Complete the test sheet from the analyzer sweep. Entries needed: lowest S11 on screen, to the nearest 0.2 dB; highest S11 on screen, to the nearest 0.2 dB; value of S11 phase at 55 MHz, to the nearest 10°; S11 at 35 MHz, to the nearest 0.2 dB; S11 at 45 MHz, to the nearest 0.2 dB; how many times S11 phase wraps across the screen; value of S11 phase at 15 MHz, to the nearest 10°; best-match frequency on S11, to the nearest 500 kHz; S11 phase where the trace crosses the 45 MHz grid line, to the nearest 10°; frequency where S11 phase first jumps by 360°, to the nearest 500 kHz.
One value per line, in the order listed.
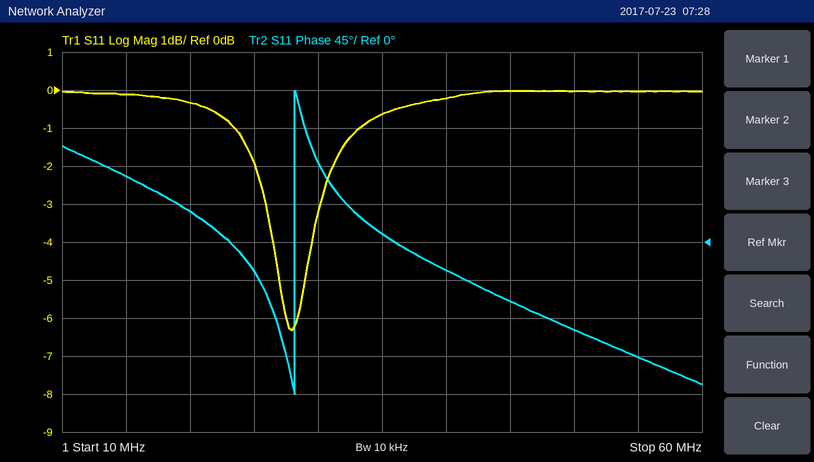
-6.4 dB
0.0 dB
-140°
-0.6 dB
0.0 dB
1
80°
28.0 MHz
-70°
28.0 MHz
